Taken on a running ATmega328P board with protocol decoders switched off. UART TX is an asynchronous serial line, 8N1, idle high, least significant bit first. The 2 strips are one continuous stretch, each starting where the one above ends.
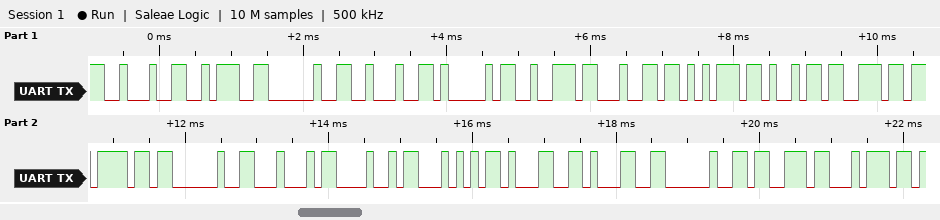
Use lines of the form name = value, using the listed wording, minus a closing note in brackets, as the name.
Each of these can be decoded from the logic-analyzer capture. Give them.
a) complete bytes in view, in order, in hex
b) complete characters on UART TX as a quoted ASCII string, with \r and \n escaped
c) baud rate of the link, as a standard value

complete bytes in view, in order, in hex = 22 3A 20 22 41 72 64 75 69 6E 6F 20 44 48 54 31 31 20 73 74
complete characters on UART TX as a quoted ASCII string, with \r and \n escaped = "\": \"Arduino DHT11 st"
baud rate of the link, as a standard value = 9600 baud
